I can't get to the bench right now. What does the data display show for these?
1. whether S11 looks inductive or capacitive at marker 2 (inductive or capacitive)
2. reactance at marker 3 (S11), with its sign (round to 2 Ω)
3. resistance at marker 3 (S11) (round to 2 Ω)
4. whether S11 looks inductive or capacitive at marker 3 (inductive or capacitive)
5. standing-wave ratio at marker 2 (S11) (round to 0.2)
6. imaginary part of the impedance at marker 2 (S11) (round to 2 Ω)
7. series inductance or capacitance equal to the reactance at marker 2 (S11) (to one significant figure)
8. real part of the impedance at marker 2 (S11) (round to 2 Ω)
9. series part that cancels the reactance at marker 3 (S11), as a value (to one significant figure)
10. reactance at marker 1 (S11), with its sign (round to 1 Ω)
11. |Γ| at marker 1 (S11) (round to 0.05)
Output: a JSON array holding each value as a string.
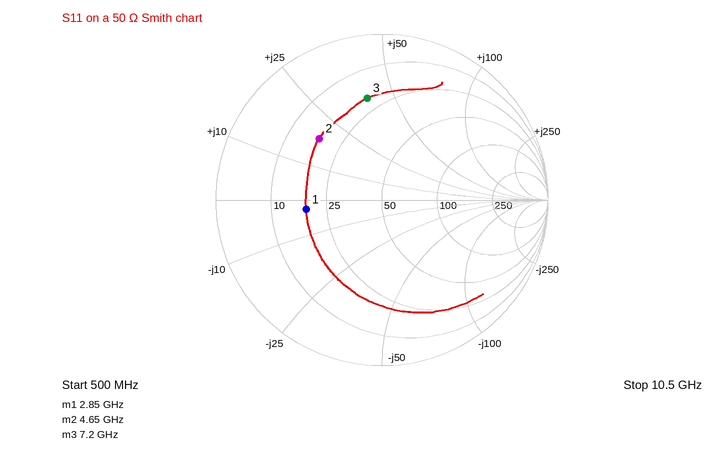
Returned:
["inductive", "+40 Ω", "20 Ω", "inductive", "3.2", "+18 Ω", "600 pH", "18 Ω", "600 fF", "-3 Ω", "0.45"]
